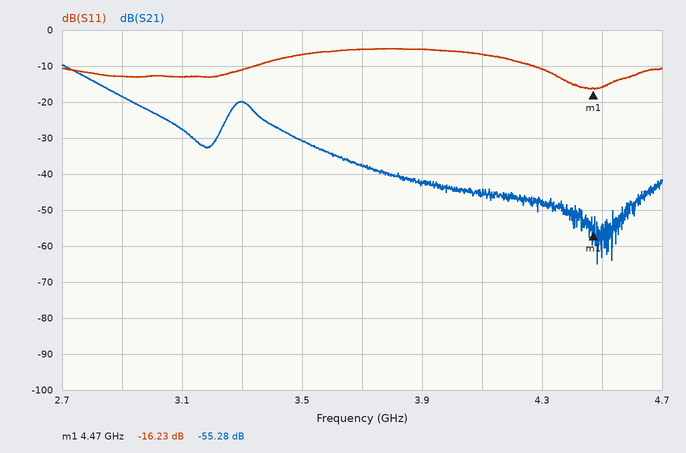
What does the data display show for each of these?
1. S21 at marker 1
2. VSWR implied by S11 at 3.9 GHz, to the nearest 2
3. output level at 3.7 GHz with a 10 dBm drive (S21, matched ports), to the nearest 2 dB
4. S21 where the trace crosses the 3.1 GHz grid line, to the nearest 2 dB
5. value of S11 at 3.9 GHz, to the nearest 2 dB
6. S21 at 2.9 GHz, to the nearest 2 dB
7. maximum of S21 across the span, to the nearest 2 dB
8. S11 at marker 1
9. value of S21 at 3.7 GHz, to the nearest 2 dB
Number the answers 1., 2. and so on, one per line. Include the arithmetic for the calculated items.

1. -55.28 dB
2. |Γ| = 10^(-6/20) = 0.5012; VSWR = (1 + 0.5012)/(1 − 0.5012) ≈ 3.01, so 4 to the nearest 2
3. 10 dBm + (-38 dB) = -28 dBm
4. -28 dB
5. -6 dB
6. -18 dB
7. -10 dB
8. -16.23 dB
9. -38 dB
